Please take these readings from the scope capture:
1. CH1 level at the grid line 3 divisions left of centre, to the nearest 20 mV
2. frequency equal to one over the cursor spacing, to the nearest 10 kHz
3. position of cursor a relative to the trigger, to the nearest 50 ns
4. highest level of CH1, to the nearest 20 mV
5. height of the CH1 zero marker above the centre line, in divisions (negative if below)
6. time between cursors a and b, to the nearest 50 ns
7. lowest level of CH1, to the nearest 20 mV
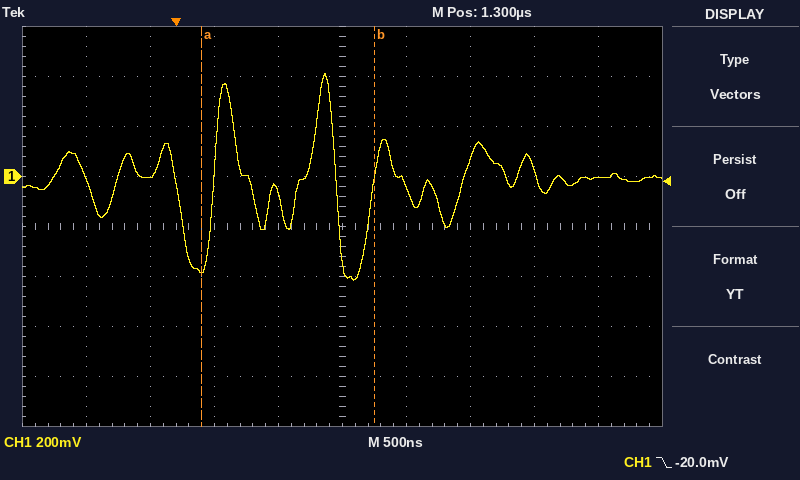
0 mV
740 kHz
+200 ns
420 mV
+1.0 div
1.35 µs
-420 mV
